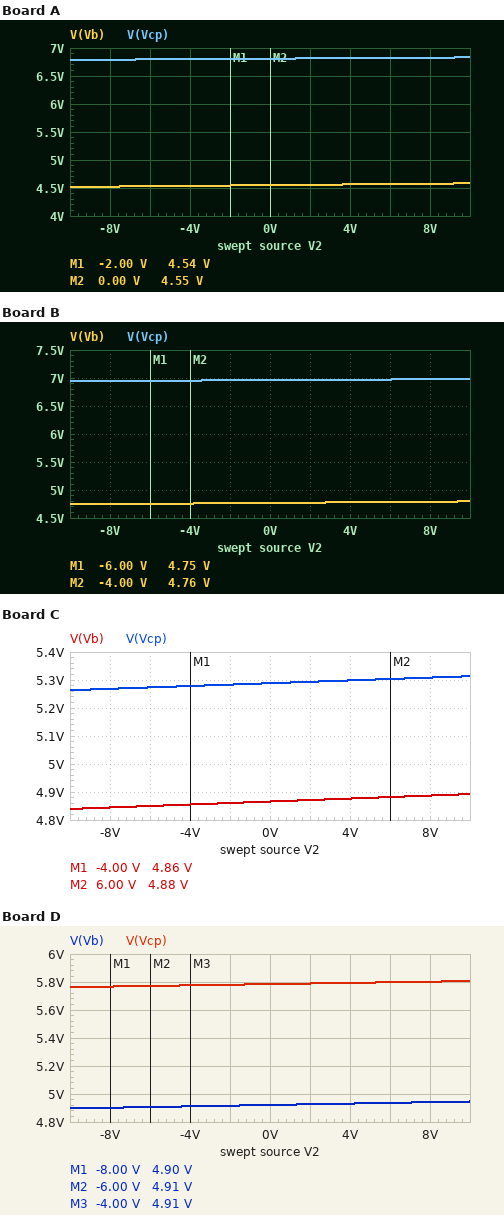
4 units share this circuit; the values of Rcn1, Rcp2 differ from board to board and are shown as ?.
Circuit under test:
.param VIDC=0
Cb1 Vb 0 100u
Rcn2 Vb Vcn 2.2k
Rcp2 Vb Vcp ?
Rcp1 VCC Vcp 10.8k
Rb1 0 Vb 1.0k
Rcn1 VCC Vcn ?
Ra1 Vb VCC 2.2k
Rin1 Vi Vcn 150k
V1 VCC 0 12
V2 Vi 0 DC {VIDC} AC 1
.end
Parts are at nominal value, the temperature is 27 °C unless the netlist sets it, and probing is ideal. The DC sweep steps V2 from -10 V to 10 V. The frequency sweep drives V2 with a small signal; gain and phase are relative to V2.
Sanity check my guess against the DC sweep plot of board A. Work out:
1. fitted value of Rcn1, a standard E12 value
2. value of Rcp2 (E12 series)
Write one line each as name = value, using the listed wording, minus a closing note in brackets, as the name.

fitted value of Rcn1, a standard E12 value = 8.2 kΩ
value of Rcp2 = 4.7 kΩ
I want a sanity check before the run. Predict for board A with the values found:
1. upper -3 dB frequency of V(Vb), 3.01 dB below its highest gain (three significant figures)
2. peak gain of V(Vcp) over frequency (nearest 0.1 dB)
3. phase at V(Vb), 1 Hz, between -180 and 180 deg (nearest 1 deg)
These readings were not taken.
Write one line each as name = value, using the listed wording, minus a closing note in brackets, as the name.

upper -3 dB frequency of V(Vb), 3.01 dB below its highest gain = 2.58 Hz
peak gain of V(Vcp) over frequency = -53.0 dB
phase at V(Vb), 1 Hz, between -180 and 180 deg = -21 deg
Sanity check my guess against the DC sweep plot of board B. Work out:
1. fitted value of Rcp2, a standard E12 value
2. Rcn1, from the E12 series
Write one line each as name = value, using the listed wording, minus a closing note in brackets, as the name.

fitted value of Rcp2, a standard E12 value = 4.7 kΩ
Rcn1, from the E12 series = 4.7 kΩ
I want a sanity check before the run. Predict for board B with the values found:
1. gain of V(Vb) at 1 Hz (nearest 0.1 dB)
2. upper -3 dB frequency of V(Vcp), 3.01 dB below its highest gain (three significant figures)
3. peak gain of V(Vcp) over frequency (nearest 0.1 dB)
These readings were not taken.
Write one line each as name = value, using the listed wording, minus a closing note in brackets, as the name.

gain of V(Vb) at 1 Hz = -52.0 dB
upper -3 dB frequency of V(Vcp), 3.01 dB below its highest gain = 2.65 Hz
peak gain of V(Vcp) over frequency = -54.5 dB
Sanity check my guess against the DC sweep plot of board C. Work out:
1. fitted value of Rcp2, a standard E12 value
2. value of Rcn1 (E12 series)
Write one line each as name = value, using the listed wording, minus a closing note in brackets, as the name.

fitted value of Rcp2, a standard E12 value = 680 Ω
value of Rcn1 = 4.7 kΩ
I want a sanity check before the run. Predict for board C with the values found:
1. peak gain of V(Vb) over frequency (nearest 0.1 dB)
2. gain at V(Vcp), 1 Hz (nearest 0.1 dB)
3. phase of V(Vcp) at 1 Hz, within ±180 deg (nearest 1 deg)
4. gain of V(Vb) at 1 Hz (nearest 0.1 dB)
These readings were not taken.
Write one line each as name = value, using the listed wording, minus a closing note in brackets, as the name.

peak gain of V(Vb) over frequency = -51.5 dB
gain at V(Vcp), 1 Hz = -52.6 dB
phase of V(Vcp) at 1 Hz, within ±180 deg = -20 deg
gain of V(Vb) at 1 Hz = -52.1 dB
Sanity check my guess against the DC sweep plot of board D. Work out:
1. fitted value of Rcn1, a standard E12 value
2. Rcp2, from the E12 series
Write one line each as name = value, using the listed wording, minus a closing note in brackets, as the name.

fitted value of Rcn1, a standard E12 value = 3.9 kΩ
Rcp2, from the E12 series = 1.5 kΩ
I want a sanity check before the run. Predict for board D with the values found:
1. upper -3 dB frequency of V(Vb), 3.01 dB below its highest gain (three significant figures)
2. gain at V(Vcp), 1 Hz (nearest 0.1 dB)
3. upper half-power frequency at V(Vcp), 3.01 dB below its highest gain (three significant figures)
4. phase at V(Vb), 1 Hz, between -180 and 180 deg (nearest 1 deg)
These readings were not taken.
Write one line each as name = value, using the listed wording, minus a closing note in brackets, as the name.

upper -3 dB frequency of V(Vb), 3.01 dB below its highest gain = 2.71 Hz
gain at V(Vcp), 1 Hz = -53.8 dB
upper half-power frequency at V(Vcp), 3.01 dB below its highest gain = 2.71 Hz
phase at V(Vb), 1 Hz, between -180 and 180 deg = -20 deg
